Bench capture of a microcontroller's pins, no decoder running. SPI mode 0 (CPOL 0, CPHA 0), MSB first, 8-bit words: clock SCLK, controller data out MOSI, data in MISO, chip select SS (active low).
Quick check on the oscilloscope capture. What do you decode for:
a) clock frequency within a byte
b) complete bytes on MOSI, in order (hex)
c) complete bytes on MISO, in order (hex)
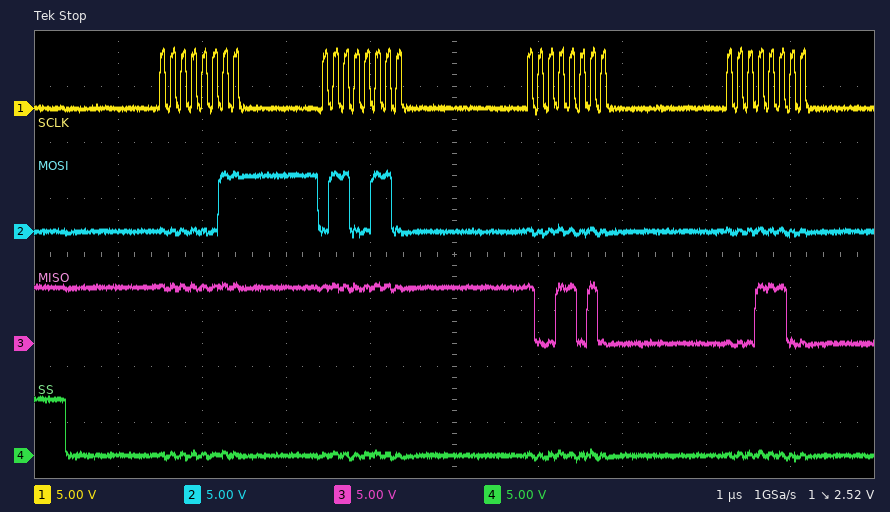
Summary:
8 MHz
03 66 00 00
FF FF 9A 1C
